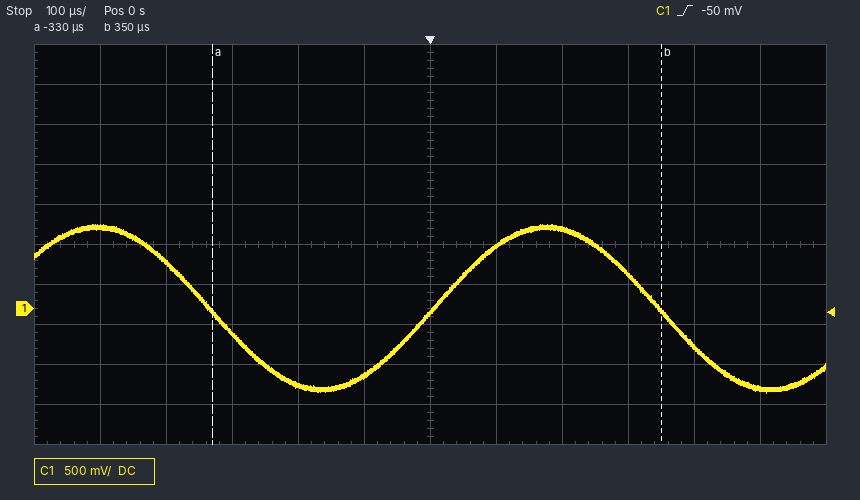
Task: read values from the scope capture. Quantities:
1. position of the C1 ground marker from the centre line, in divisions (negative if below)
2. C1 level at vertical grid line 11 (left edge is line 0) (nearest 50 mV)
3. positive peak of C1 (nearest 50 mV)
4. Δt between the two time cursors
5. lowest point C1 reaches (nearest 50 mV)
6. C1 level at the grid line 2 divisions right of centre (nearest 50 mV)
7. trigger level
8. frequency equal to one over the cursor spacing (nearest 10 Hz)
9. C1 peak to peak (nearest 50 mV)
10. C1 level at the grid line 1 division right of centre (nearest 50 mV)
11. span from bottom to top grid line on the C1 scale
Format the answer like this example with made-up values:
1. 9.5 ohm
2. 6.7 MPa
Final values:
1. -1.6 div
2. -1.00 V
3. 1.05 V
4. 680 µs
5. -1.05 V
6. 1.00 V
7. -50 mV
8. 1.47 kHz
9. 2.10 V
10. 800 mV
11. 5 V
